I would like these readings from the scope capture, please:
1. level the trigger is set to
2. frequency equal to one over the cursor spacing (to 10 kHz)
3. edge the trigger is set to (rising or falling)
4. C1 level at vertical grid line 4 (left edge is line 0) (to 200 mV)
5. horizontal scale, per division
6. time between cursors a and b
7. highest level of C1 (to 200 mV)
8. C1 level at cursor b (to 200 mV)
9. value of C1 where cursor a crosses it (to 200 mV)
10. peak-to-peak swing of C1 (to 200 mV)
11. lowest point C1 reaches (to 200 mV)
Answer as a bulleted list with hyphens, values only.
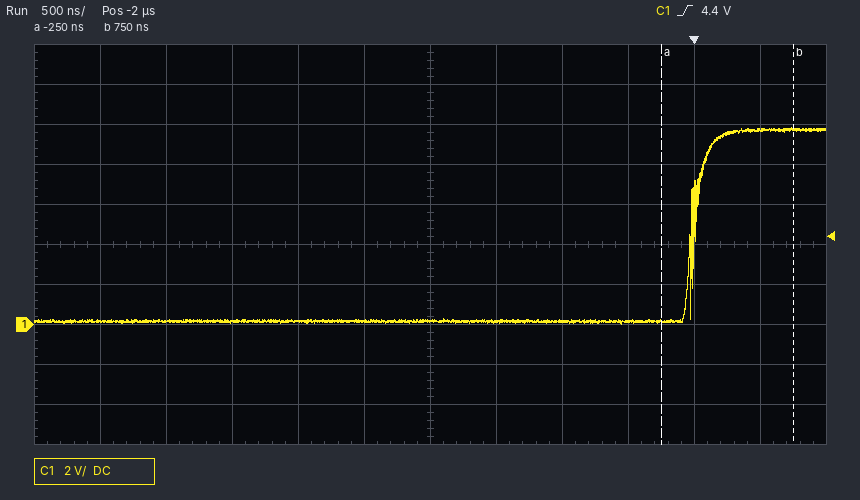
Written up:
- 4.4 V
- 1.00 MHz
- rising
- 200 mV
- 500 ns
- 1.00 µs
- 9.8 V
- 9.8 V
- 200 mV
- 9.8 V
- 0.0 V
